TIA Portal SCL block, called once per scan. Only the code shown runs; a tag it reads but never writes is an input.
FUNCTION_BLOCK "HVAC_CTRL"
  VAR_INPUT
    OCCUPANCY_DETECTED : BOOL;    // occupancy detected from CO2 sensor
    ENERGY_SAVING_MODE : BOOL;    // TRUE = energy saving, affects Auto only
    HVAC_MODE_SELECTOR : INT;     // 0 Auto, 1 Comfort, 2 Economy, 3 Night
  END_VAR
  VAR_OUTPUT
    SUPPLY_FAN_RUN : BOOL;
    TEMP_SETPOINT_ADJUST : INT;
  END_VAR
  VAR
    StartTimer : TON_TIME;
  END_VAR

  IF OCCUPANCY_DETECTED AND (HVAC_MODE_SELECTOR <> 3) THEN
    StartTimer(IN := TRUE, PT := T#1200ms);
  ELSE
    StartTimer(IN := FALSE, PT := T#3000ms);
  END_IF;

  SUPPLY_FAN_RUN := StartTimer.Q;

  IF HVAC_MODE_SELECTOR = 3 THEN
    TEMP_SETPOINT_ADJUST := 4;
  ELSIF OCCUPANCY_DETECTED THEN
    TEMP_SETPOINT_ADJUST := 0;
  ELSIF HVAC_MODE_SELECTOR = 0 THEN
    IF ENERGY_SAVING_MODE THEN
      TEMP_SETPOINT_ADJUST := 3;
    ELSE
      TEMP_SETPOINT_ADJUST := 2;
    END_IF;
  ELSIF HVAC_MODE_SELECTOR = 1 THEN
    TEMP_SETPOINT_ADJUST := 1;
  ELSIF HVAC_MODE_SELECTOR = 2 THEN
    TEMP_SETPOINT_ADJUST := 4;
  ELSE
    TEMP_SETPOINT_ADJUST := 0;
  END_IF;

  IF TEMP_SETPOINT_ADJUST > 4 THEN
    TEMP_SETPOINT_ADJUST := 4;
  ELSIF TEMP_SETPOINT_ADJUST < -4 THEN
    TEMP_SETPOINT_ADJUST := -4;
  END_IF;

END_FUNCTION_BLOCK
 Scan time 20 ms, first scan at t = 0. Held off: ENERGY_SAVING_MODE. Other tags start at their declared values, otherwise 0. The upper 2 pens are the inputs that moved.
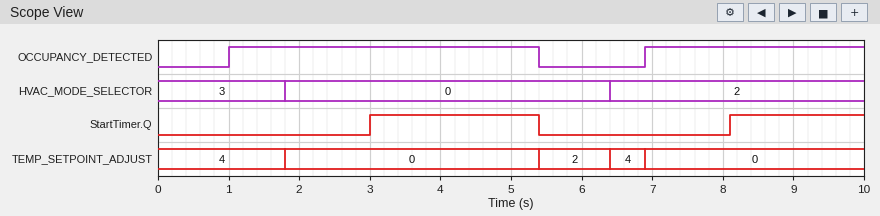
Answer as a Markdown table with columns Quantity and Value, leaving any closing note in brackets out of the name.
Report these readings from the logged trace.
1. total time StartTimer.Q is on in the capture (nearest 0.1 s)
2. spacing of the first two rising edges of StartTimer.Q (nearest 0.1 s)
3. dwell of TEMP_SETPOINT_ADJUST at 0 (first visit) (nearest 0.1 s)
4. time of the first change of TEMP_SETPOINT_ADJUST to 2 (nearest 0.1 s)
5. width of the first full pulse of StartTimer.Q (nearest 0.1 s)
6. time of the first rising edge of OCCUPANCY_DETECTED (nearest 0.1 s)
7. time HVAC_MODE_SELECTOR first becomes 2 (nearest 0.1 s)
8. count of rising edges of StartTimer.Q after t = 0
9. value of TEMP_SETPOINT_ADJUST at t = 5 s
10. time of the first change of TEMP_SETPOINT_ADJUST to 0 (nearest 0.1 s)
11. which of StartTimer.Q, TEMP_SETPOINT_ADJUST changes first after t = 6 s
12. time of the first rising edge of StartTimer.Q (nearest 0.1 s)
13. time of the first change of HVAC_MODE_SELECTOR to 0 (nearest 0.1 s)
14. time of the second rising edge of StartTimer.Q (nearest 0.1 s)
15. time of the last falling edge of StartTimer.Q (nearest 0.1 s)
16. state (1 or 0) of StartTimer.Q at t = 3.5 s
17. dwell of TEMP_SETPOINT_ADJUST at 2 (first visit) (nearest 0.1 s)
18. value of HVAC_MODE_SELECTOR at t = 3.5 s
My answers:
| Quantity | Value |
|---|---|
| total time StartTimer.Q is on in the capture | 4.3 s |
| spacing of the first two rising edges of StartTimer.Q | 5.1 s |
| dwell of TEMP_SETPOINT_ADJUST at 0 (first visit) | 3.6 s |
| time of the first change of TEMP_SETPOINT_ADJUST to 2 | 5.4 s |
| width of the first full pulse of StartTimer.Q | 2.4 s |
| time of the first rising edge of OCCUPANCY_DETECTED | 1.0 s |
| time HVAC_MODE_SELECTOR first becomes 2 | 6.4 s |
| count of rising edges of StartTimer.Q after t = 0 | 2 |
| value of TEMP_SETPOINT_ADJUST at t = 5 s | 0 |
| time of the first change of TEMP_SETPOINT_ADJUST to 0 | 1.8 s |
| which of StartTimer.Q, TEMP_SETPOINT_ADJUST changes first after t = 6 s | TEMP_SETPOINT_ADJUST |
| time of the first rising edge of StartTimer.Q | 3.0 s |
| time of the first change of HVAC_MODE_SELECTOR to 0 | 1.8 s |
| time of the second rising edge of StartTimer.Q | 8.1 s |
| time of the last falling edge of StartTimer.Q | 5.4 s |
| state (1 or 0) of StartTimer.Q at t = 3.5 s | 1 |
| dwell of TEMP_SETPOINT_ADJUST at 2 (first visit) | 1.0 s |
| value of HVAC_MODE_SELECTOR at t = 3.5 s | 0 |
